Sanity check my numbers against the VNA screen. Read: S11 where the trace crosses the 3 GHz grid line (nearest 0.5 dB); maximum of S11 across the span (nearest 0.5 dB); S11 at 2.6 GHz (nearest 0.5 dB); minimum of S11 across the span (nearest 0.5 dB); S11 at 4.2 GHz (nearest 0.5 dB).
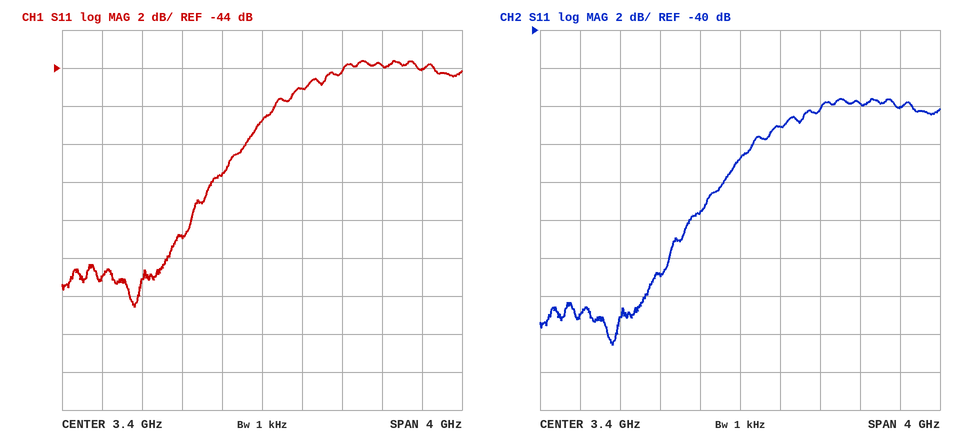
-49.5 dB
-43.5 dB
-53.0 dB
-56.5 dB
-44.0 dB
